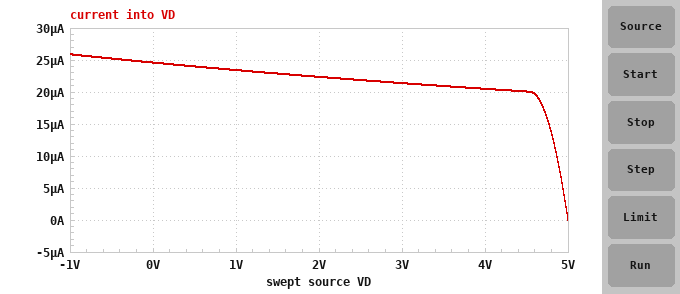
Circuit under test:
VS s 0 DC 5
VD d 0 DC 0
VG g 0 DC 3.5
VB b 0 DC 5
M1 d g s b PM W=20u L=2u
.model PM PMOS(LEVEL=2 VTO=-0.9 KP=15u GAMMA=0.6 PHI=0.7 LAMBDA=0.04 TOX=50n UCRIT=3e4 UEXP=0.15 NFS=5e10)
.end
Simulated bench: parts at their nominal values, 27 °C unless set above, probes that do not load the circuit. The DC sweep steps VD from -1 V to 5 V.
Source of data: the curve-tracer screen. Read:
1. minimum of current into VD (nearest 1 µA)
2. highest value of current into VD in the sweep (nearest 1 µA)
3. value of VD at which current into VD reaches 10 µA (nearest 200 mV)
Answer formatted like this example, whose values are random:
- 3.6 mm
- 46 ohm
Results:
- 0 A
- 26 µA
- 4.8 V
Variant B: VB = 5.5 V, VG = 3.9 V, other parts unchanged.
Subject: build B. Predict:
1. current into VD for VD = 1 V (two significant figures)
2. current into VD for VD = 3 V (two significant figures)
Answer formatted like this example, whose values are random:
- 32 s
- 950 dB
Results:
- 140 nA
- 130 nA
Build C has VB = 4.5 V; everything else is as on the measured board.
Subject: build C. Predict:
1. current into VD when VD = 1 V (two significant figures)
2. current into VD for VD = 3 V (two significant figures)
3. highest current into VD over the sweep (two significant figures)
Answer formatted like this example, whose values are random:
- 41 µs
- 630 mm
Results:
- 48 µA
- 44 µA
- 53 µA
